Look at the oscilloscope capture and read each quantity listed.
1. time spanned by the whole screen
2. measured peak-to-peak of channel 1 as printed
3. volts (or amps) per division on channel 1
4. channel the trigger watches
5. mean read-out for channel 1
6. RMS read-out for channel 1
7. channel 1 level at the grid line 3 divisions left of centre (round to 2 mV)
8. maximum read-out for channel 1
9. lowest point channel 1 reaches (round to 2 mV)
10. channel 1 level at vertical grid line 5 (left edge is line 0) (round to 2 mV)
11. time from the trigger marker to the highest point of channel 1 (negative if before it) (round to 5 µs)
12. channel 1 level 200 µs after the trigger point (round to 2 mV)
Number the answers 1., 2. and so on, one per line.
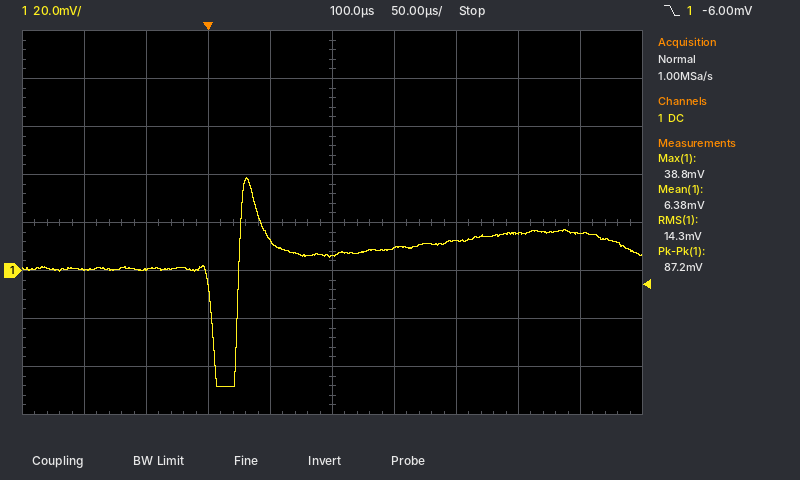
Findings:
1. 500 µs
2. 87.2 mV
3. 20 mV
4. channel 1
5. 6.38 mV
6. 14.3 mV
7. 0 mV
8. 38.8 mV
9. -48 mV
10. 6 mV
11. +30 µs
12. 12 mV
